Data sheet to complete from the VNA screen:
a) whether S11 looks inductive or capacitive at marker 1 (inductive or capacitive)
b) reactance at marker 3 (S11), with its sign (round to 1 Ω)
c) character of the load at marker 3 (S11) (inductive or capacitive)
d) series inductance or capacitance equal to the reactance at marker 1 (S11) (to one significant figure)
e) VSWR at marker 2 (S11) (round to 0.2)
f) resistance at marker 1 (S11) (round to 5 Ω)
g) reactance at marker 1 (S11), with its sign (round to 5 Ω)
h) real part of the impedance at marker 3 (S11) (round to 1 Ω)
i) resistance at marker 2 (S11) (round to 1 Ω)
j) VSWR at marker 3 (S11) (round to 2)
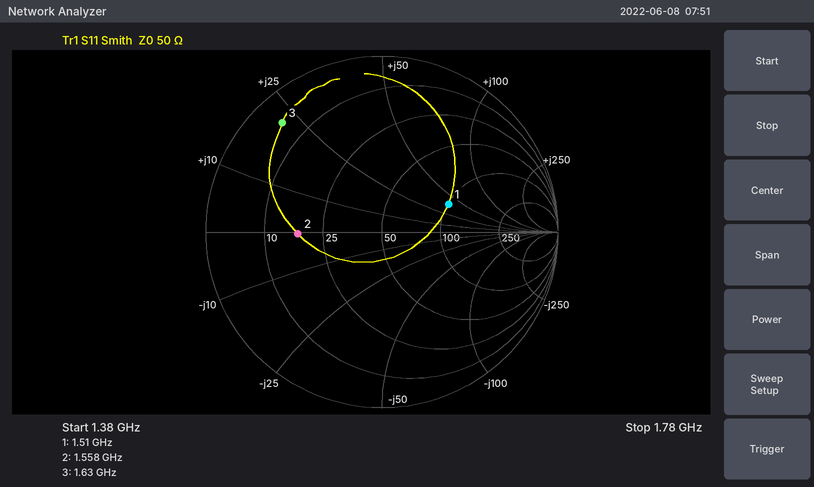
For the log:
inductive
+22 Ω
inductive
4 nH
2.8
100 Ω
+40 Ω
5 Ω
18 Ω
12
